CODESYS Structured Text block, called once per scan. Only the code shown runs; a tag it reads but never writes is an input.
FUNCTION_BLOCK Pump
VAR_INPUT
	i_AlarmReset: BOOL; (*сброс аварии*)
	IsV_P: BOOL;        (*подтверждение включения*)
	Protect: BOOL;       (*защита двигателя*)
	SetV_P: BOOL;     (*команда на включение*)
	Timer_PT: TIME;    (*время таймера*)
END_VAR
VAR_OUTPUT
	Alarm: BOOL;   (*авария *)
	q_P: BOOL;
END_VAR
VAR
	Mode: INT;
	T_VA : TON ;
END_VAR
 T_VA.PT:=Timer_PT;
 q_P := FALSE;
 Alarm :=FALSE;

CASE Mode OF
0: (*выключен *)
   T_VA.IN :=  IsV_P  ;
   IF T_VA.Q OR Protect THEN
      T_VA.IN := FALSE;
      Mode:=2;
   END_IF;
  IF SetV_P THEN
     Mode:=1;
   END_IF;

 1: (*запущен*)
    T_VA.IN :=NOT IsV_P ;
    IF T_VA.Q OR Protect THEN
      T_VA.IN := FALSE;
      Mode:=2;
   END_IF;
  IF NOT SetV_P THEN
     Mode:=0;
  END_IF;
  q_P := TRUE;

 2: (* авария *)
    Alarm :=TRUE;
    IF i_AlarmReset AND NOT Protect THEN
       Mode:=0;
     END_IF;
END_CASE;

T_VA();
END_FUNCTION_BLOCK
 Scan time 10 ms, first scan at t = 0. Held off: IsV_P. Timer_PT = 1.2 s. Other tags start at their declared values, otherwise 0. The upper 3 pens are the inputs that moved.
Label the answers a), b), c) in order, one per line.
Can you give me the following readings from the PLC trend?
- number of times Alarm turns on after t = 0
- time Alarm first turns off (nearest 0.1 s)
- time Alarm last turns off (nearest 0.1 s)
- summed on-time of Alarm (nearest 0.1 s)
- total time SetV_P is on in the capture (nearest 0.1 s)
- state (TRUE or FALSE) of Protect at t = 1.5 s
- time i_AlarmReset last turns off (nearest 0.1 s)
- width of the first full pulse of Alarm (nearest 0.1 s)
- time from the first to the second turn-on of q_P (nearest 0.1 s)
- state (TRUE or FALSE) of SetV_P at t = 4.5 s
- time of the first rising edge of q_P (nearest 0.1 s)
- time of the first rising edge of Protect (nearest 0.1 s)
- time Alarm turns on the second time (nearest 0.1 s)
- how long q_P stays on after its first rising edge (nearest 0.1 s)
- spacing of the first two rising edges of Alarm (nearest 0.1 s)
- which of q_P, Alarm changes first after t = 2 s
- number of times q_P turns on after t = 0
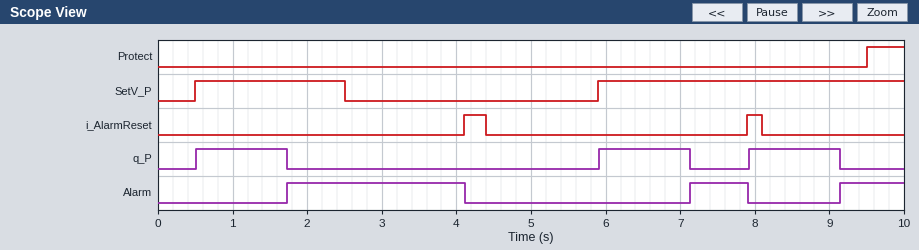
a) 3
b) 4.1 s
c) 7.9 s
d) 4.0 s
e) 6.1 s
f) FALSE
g) 8.1 s
h) 2.4 s
i) 5.4 s
j) FALSE
k) 0.5 s
l) 9.5 s
m) 7.1 s
n) 1.2 s
o) 5.4 s
p) Alarm
q) 3
